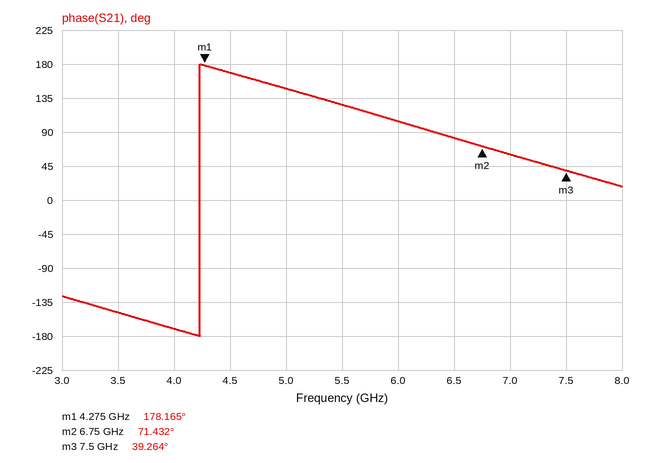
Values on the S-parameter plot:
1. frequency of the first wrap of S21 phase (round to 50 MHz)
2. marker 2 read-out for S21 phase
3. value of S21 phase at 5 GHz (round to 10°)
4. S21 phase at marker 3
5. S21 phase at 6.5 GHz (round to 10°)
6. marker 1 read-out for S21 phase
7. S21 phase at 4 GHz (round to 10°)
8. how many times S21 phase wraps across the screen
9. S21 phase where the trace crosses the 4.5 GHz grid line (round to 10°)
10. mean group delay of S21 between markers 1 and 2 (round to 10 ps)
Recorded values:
4.25 GHz
71.432°
150°
39.264°
80°
178.165°
-170°
1
170°
120 ps
